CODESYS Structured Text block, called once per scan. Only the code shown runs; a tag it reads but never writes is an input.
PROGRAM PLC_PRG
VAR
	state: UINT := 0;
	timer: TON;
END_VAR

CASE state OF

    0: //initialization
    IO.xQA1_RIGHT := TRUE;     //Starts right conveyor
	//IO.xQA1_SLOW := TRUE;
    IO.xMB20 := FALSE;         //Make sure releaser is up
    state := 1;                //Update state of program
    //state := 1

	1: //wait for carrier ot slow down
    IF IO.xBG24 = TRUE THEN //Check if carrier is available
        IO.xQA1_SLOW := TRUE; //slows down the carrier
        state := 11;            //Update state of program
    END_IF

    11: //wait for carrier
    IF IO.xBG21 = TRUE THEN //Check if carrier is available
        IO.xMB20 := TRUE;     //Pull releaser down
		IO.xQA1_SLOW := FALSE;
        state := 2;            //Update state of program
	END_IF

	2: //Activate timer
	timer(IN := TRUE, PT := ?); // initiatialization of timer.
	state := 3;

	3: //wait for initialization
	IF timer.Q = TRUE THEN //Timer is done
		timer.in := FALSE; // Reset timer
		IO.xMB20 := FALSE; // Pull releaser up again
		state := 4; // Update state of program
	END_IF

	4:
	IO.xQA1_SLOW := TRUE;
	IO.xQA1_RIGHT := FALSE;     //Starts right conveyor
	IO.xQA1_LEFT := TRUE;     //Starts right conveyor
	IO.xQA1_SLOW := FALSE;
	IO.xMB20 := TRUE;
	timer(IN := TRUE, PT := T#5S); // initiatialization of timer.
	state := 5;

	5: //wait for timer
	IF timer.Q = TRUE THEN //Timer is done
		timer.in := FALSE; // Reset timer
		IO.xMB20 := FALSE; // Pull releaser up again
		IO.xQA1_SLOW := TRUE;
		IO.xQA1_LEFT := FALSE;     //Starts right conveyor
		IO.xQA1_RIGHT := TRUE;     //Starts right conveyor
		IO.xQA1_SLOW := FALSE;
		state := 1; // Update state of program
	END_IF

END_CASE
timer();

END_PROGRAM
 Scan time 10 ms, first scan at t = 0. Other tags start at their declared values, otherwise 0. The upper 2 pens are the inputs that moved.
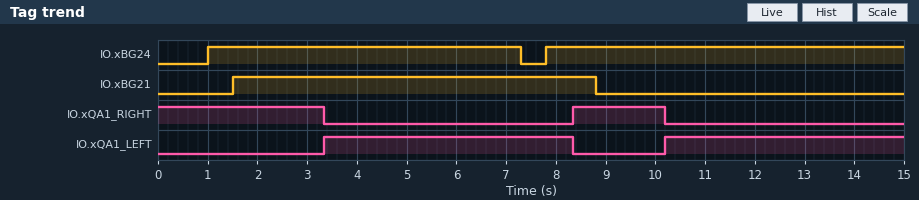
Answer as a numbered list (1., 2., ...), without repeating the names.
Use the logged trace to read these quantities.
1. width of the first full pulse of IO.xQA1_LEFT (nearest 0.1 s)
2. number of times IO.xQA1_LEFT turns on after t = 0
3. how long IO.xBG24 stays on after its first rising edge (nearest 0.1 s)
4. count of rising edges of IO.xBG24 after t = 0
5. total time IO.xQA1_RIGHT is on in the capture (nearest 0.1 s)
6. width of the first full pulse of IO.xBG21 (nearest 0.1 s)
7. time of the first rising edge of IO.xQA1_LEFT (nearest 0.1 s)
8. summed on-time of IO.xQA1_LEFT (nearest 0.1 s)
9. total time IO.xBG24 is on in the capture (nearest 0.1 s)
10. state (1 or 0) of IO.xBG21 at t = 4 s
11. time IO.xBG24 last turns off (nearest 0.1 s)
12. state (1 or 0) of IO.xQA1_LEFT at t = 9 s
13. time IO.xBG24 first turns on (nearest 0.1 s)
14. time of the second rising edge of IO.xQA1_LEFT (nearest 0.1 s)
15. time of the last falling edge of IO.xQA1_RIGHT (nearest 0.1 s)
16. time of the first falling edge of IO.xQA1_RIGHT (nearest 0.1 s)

1. 5.0 s
2. 2
3. 6.3 s
4. 2
5. 5.2 s
6. 7.3 s
7. 3.3 s
8. 9.8 s
9. 13.5 s
10. 1
11. 7.3 s
12. 0
13. 1.0 s
14. 10.2 s
15. 10.2 s
16. 3.3 s
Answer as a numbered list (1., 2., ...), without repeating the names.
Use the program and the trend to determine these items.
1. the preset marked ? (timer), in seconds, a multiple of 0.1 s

1. 1.8 s
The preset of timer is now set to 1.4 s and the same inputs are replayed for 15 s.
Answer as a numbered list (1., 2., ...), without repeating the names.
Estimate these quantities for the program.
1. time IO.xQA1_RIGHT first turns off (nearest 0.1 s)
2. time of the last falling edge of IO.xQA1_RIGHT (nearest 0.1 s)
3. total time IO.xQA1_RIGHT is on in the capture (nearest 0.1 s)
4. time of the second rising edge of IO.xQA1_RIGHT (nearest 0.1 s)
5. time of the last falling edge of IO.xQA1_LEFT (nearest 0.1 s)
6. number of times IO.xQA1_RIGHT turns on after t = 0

1. 2.9 s
2. 9.4 s
3. 5.0 s
4. 14.4 s
5. 14.4 s
6. 2
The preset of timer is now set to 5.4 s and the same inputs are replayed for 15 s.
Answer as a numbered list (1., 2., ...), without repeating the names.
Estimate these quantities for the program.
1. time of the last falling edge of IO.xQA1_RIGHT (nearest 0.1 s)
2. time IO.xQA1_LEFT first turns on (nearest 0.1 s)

1. 6.9 s
2. 6.9 s
